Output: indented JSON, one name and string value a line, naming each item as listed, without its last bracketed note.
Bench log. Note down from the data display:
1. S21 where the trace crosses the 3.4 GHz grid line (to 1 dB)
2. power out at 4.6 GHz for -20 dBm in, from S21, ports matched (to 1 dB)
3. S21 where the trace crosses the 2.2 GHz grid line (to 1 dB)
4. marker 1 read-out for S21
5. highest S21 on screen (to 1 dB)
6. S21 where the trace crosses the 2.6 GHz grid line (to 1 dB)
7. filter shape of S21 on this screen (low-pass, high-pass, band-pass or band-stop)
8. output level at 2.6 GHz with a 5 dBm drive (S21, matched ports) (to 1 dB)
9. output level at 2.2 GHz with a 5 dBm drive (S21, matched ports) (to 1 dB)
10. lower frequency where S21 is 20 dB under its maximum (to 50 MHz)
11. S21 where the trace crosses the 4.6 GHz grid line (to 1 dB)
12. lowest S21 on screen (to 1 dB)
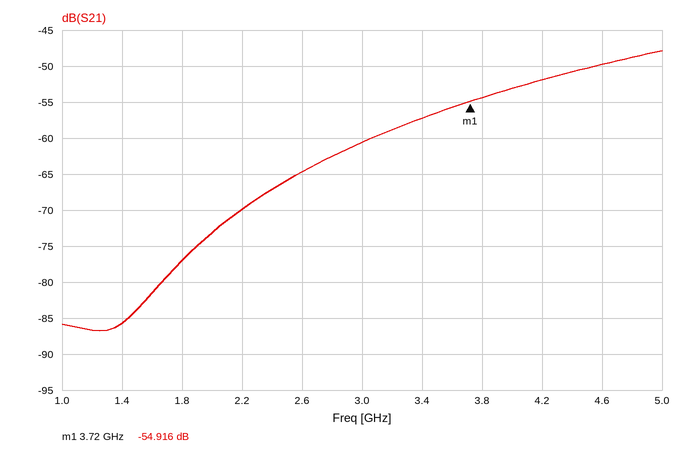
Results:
{
  "S21 where the trace crosses the 3.4 GHz grid line": "-57 dB",
  "power out at 4.6 GHz for -20 dBm in, from S21, ports matched": "-70 dBm",
  "S21 where the trace crosses the 2.2 GHz grid line": "-70 dB",
  "marker 1 read-out for S21": "-54.916 dB",
  "highest S21 on screen": "-48 dB",
  "S21 where the trace crosses the 2.6 GHz grid line": "-65 dB",
  "filter shape of S21 on this screen": "high-pass",
  "output level at 2.6 GHz with a 5 dBm drive (S21, matched ports)": "-60 dBm",
  "output level at 2.2 GHz with a 5 dBm drive (S21, matched ports)": "-65 dBm",
  "lower frequency where S21 is 20 dB under its maximum": "2.35 GHz",
  "S21 where the trace crosses the 4.6 GHz grid line": "-50 dB",
  "lowest S21 on screen": "-87 dB"
}
